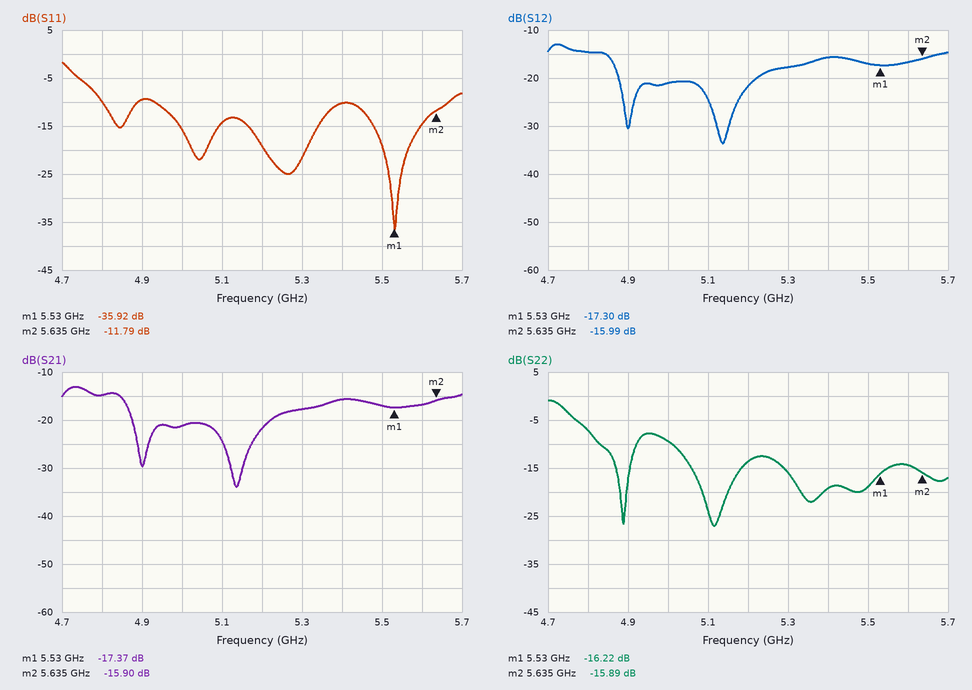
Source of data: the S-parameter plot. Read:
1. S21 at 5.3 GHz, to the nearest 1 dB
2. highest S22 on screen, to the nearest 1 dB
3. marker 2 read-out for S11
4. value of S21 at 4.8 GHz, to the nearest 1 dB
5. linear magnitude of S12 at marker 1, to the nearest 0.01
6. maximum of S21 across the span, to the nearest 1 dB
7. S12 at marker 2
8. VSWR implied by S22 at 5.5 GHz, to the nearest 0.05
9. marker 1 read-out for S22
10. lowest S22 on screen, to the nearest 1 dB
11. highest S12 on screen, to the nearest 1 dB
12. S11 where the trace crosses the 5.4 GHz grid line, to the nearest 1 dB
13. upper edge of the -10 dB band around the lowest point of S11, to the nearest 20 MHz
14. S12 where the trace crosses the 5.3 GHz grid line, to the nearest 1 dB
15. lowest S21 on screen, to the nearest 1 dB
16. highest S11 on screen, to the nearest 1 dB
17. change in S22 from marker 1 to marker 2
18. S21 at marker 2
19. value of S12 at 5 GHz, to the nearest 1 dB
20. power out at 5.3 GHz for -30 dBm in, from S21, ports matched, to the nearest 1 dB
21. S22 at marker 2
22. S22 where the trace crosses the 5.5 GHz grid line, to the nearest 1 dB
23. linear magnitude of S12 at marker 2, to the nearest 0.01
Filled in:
-18 dB
-1 dB
-11.79 dB
-15 dB
0.14
-13 dB
-15.99 dB
1.25
-16.22 dB
-27 dB
-13 dB
-10 dB
5.66 GHz
-18 dB
-34 dB
-2 dB
0.33 dB
-15.90 dB
-21 dB
-48 dBm
-15.89 dB
-19 dB
0.16
